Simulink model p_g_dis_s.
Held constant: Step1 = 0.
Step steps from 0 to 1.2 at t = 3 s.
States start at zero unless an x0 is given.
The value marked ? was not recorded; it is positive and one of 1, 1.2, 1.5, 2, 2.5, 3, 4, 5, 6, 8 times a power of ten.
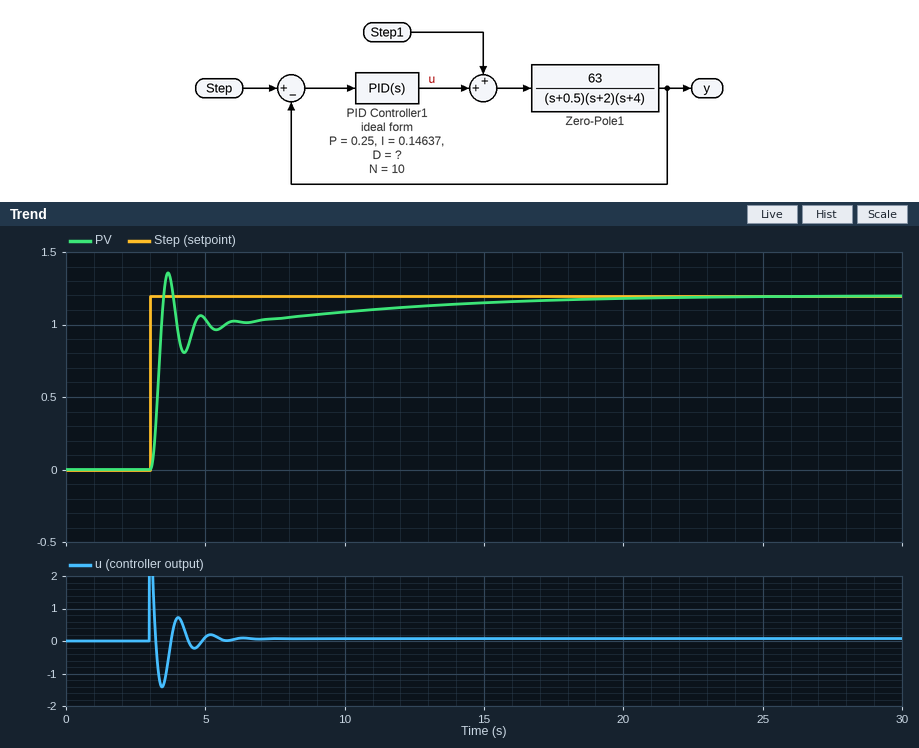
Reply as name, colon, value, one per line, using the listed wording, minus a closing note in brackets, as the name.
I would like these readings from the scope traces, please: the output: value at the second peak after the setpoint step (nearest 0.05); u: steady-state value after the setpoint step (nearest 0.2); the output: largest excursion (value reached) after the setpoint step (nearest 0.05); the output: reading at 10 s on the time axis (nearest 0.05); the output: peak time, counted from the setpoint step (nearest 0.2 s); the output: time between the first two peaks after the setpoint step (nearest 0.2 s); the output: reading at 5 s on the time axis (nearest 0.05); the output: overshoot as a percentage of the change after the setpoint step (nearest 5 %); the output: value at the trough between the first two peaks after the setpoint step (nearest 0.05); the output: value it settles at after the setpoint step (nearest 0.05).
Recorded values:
the output: value at the second peak after the setpoint step: 1.05
u: steady-state value after the setpoint step: 0.0
the output: largest excursion (value reached) after the setpoint step: 1.35
the output: reading at 10 s on the time axis: 1.10
the output: peak time, counted from the setpoint step: 0.6 s
the output: time between the first two peaks after the setpoint step: 1.2 s
the output: reading at 5 s on the time axis: 1.05
the output: overshoot as a percentage of the change after the setpoint step: 15 %
the output: value at the trough between the first two peaks after the setpoint step: 0.80
the output: value it settles at after the setpoint step: 1.20
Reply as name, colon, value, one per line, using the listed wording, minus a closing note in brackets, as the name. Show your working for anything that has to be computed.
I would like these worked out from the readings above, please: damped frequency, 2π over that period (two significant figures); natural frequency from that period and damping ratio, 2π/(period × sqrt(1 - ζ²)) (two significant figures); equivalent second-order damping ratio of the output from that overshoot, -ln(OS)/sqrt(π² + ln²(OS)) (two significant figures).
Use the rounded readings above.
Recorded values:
damped frequency, 2π over that period: 2π / 1.2 = 5.2 rad/s
natural frequency from that period and damping ratio, 2π/(period × sqrt(1 - ζ²)): 2π / (1.2 × sqrt(1 - 0.52²)) = 6.1 rad/s
equivalent second-order damping ratio of the output from that overshoot, -ln(OS)/sqrt(π² + ln²(OS)): ln(0.15) = -1.897; 1.897 / sqrt(9.870 + 3.599) = 0.52
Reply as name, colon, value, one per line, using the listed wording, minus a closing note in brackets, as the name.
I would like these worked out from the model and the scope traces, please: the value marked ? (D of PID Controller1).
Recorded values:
the value marked ?: 2
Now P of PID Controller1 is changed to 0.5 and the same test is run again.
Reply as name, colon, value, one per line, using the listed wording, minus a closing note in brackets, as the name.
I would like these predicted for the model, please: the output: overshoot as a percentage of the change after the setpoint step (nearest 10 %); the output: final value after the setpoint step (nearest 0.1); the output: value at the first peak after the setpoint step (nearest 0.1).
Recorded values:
the output: overshoot as a percentage of the change after the setpoint step: 50 %
the output: final value after the setpoint step: 1.2
the output: value at the first peak after the setpoint step: 1.8
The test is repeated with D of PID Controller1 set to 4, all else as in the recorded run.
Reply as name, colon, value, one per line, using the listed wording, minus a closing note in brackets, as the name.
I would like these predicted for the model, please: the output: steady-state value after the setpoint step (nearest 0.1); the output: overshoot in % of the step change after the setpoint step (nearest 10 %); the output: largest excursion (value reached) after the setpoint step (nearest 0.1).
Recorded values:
the output: steady-state value after the setpoint step: 1.2
the output: overshoot in % of the step change after the setpoint step: 40 %
the output: largest excursion (value reached) after the setpoint step: 1.7
